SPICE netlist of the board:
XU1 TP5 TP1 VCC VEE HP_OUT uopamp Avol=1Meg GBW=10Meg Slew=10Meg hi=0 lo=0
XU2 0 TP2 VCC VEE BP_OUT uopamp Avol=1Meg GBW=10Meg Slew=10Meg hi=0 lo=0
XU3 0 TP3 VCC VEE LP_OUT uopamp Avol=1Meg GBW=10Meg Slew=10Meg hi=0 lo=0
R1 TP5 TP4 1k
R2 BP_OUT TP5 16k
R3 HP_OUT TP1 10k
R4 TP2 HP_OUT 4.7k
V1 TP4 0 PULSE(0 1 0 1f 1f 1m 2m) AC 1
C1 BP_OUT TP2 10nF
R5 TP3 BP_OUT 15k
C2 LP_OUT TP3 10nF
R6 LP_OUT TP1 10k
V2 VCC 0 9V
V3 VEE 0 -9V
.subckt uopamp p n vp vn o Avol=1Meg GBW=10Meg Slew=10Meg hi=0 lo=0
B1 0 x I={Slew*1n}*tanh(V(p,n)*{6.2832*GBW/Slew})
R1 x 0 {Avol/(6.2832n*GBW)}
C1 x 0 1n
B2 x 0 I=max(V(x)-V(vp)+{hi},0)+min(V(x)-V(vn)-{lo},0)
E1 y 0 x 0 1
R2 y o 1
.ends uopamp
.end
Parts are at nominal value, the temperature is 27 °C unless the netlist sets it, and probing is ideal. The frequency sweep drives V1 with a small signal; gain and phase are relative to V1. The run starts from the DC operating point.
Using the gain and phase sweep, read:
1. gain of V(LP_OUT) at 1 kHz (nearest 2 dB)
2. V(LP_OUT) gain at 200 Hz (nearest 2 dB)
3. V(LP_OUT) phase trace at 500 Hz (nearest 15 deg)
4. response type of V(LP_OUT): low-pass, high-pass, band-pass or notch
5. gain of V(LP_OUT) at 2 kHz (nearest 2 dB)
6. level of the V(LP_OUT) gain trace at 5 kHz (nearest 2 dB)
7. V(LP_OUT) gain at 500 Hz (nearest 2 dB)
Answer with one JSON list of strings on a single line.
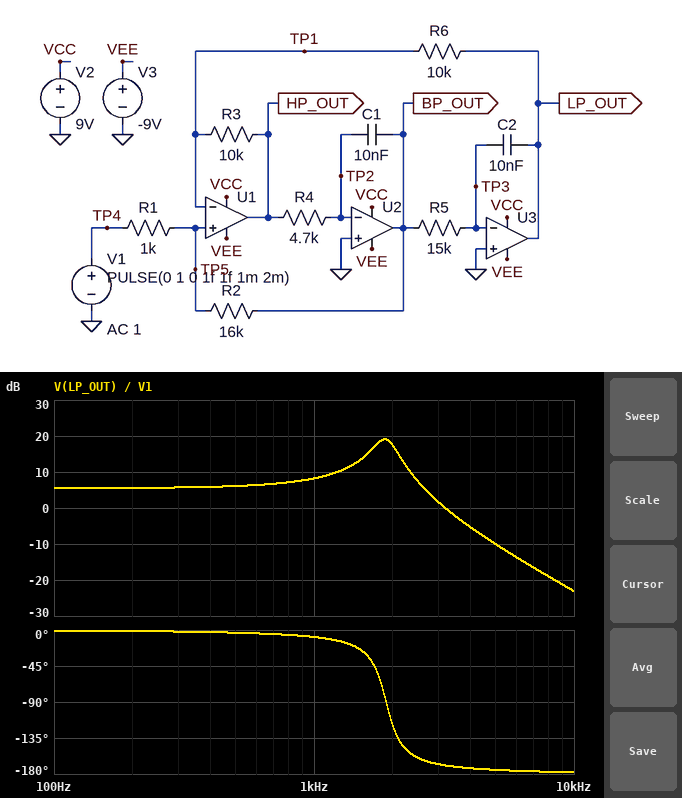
["8 dB", "6 dB", "0 deg", "low-pass", "18 dB", "-10 dB", "6 dB"]
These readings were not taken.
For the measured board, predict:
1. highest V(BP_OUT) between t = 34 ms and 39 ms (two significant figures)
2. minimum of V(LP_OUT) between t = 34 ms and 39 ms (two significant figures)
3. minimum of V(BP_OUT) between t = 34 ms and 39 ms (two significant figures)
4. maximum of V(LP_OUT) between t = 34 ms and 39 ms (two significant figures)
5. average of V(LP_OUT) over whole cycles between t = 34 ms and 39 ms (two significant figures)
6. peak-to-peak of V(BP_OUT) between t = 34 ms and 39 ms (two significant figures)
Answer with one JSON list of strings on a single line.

["2.4 V", "-1.1 V", "-2.4 V", "3.0 V", "940 mV", "4.8 V"]
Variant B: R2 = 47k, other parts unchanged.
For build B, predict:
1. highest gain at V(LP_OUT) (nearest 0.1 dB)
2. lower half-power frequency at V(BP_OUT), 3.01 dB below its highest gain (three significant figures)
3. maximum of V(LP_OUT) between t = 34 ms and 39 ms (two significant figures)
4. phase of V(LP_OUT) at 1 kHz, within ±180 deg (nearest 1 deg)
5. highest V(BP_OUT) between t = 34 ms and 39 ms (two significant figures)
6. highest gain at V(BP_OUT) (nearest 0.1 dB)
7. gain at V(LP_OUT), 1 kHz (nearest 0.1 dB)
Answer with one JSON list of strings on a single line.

["28.5 dB", "1.83 kHz", "3.1 V", "-3 deg", "2.1 V", "33.5 dB", "8.7 dB"]
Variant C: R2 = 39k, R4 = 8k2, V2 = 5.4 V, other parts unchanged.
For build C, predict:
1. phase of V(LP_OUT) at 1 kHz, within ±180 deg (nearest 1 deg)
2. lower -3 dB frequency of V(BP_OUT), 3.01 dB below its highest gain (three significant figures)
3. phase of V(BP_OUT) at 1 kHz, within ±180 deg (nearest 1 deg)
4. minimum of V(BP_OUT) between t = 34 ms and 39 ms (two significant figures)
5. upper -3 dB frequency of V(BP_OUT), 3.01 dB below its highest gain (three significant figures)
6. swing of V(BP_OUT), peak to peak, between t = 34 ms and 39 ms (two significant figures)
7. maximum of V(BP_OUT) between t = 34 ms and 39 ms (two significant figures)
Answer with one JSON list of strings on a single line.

["-5 deg", "1.39 kHz", "-95 deg", "-5.4 V", "1.48 kHz", "11 V", "5.3 V"]
